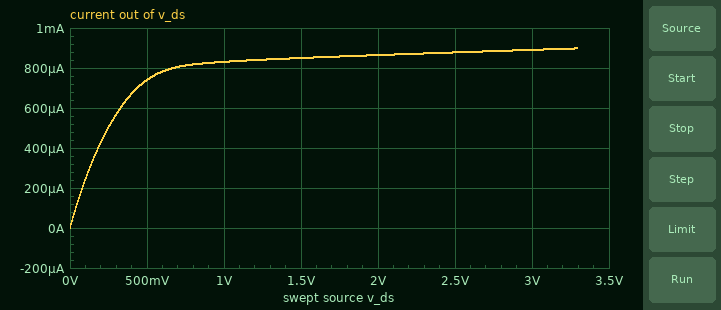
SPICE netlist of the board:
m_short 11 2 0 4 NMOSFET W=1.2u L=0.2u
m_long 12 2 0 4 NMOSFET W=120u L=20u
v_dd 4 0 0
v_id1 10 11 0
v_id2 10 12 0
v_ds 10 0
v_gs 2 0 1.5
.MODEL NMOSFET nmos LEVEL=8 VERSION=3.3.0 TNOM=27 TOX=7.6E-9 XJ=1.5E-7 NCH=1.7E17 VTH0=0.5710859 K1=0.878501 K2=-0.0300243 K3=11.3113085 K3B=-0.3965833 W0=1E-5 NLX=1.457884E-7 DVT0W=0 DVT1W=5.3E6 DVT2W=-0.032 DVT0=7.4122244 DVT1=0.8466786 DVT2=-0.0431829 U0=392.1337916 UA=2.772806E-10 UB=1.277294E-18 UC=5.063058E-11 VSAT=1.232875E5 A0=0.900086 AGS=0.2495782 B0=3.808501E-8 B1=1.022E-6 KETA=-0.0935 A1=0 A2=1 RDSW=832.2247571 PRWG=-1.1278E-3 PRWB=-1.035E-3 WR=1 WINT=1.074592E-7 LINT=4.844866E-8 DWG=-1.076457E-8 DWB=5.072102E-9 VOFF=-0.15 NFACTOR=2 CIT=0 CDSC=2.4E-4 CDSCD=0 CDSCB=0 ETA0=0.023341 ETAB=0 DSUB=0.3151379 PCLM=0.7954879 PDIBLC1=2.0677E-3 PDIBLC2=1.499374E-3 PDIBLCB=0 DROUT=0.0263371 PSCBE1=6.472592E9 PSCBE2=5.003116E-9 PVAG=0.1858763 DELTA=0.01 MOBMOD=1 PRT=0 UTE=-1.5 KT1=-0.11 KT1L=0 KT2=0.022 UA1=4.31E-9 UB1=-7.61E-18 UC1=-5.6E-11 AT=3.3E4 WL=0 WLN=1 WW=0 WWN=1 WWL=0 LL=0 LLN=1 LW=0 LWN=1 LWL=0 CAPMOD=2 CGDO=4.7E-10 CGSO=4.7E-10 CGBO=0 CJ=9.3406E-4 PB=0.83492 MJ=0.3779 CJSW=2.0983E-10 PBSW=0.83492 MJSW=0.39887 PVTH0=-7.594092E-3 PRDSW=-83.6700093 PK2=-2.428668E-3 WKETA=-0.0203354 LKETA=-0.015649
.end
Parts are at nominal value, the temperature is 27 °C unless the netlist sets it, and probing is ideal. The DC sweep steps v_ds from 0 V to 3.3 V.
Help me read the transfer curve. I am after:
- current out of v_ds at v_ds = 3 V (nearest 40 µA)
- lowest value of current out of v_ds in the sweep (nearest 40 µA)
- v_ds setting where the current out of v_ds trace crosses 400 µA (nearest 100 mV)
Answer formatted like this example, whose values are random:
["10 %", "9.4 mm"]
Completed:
["880 µA", "0 A", "200 mV"]
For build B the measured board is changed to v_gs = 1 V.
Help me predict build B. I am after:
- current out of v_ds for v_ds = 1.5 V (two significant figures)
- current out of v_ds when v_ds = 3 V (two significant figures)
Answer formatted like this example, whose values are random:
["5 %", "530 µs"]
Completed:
["370 µA", "410 µA"]
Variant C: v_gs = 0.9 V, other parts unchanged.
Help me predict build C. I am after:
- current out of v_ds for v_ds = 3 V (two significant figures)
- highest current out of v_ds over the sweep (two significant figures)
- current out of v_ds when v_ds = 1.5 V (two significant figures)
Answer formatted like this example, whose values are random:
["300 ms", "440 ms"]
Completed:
["330 µA", "340 µA", "300 µA"]
